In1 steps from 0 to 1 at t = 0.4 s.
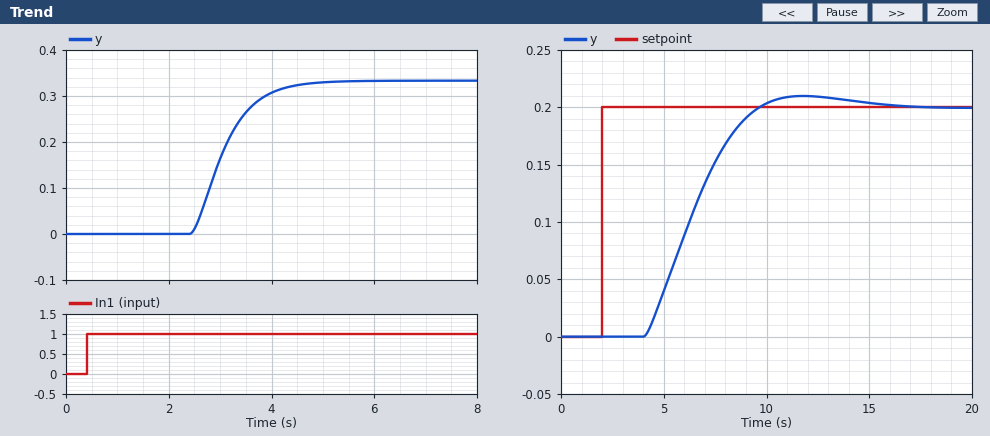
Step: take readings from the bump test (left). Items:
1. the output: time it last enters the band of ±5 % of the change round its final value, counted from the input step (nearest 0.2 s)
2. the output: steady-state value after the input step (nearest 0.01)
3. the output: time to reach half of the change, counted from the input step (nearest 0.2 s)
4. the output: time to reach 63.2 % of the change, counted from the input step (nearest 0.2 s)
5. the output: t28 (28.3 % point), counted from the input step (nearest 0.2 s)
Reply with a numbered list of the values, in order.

1. 3.8 s
2. 0.33
3. 2.6 s
4. 2.8 s
5. 2.4 s
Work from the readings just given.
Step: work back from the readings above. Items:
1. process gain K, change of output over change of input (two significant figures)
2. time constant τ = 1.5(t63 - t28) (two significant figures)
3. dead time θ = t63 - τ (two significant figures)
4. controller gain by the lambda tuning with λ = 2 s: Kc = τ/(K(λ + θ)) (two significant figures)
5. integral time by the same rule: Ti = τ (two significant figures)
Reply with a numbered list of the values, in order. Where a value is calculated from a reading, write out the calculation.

1. (0.33 - 0) / 1 = 0.33
2. 1.5 × (2.8 - 2.4) = 0.60 s
3. 2.8 - 0.6 = 2.2 s
4. 0.6 / (0.33 × (2 + 2.2)) = 0.43
5. 0.60 s
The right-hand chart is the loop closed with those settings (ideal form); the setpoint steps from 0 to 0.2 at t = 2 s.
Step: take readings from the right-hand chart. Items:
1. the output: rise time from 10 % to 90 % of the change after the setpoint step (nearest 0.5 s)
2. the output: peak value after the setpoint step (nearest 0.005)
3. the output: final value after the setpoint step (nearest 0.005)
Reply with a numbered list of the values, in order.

1. 4.0 s
2. 0.210
3. 0.200
